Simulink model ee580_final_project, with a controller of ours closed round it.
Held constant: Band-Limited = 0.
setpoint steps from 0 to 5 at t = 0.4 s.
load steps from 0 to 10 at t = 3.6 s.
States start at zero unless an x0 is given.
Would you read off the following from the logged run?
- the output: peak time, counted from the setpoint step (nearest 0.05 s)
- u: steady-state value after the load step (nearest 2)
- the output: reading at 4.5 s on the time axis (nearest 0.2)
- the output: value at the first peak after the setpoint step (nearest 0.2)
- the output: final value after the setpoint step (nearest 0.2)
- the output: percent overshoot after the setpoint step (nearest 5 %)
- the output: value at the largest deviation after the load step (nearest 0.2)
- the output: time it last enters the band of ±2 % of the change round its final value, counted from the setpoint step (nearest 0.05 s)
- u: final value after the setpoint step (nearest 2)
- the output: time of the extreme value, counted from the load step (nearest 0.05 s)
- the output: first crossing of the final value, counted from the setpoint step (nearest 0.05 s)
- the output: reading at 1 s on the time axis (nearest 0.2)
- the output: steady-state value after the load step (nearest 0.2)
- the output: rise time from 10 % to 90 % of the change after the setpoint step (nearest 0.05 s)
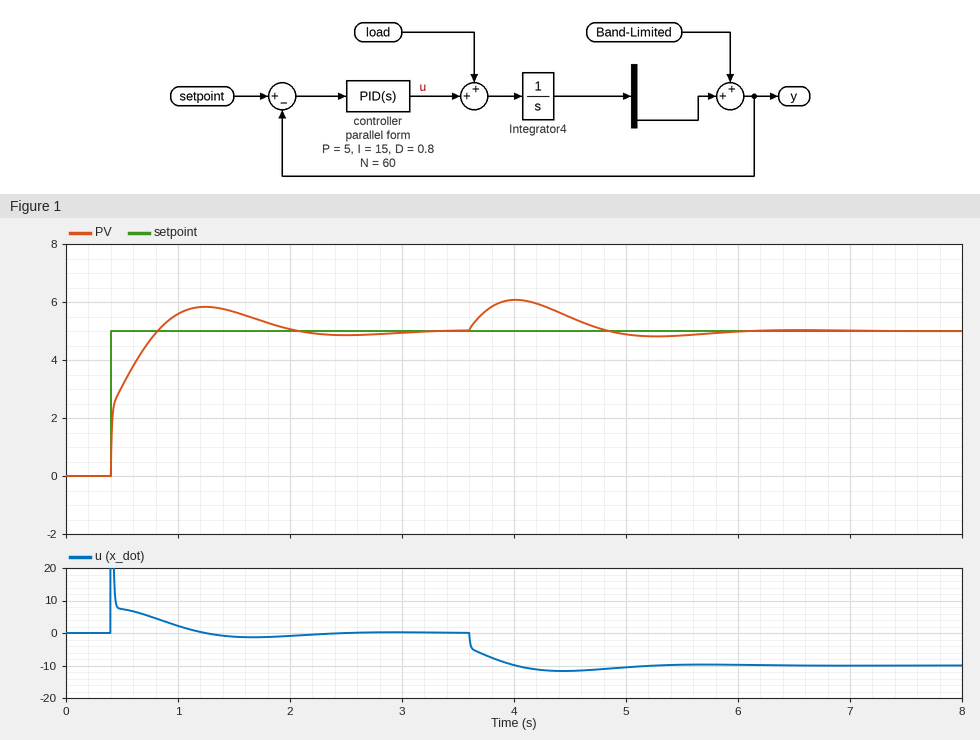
0.85 s
-10
5.4
5.8
5.0
15 %
6.0
2.45 s
0
0.40 s
0.40 s
5.6
5.0
0.30 s
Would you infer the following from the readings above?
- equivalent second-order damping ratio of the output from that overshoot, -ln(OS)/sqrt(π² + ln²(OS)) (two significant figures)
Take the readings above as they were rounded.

0.52
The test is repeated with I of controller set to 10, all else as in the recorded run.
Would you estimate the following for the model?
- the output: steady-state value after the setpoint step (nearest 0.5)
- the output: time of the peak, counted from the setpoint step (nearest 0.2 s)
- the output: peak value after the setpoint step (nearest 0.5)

5.0
1.0 s
5.5
